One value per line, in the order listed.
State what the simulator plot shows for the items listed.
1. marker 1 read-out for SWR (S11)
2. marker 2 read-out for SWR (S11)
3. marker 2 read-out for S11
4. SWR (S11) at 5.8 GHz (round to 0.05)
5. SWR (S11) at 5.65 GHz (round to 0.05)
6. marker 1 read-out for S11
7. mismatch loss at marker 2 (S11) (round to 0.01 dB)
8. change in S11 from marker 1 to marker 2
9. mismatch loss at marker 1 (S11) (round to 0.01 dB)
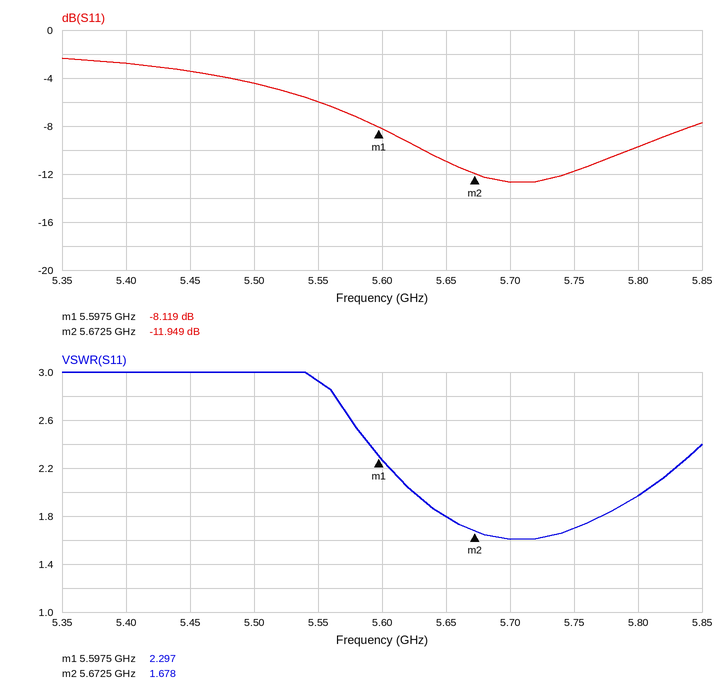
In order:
2.297
1.678
-11.949 dB
1.95
1.80
-8.119 dB
0.29 dB
-3.830 dB
0.73 dB
